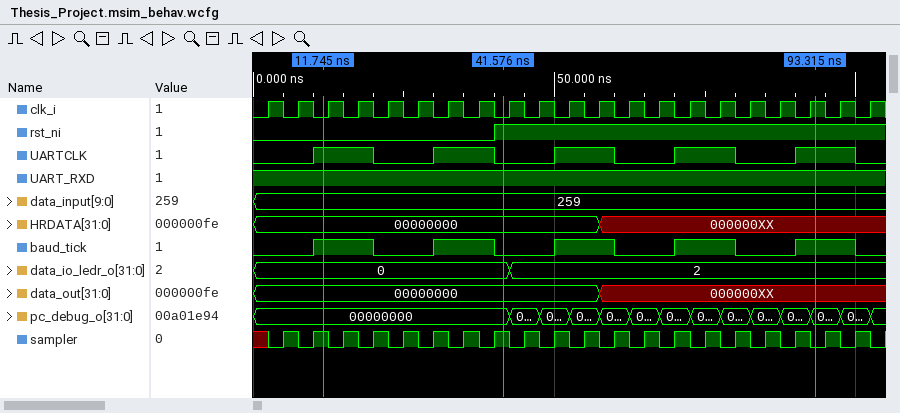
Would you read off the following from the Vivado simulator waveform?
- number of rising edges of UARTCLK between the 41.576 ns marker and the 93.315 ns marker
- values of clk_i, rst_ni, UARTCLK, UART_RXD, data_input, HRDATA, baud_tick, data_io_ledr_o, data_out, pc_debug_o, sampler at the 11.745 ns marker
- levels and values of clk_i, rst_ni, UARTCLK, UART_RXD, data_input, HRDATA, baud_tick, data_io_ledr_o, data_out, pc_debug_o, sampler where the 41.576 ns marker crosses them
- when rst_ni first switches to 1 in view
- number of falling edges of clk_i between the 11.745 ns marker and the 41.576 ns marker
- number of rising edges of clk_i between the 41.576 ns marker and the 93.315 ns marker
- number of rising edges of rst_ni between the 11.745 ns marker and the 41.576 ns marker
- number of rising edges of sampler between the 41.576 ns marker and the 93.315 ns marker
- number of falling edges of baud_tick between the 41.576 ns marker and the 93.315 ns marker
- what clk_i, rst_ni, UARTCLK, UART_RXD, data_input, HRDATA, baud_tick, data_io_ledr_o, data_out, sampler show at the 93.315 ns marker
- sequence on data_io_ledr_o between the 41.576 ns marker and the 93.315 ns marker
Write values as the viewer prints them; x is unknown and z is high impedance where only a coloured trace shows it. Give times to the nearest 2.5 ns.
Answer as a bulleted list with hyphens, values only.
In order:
- 3
- clk_i=0, rst_ni=0, UARTCLK=1, UART_RXD=1, data_input=259, HRDATA=00000000, baud_tick=1, data_io_ledr_o=0, data_out=00000000, pc_debug_o=00000000, sampler=1
- clk_i=0, rst_ni=1, UARTCLK=0, UART_RXD=1, data_input=259, HRDATA=00000000, baud_tick=0, data_io_ledr_o=0, data_out=00000000, pc_debug_o=00000000, sampler=1
- 40 ns
- 6
- 11
- 1
- 10
- 2
- clk_i=1, rst_ni=1, UARTCLK=1, UART_RXD=1, data_input=259, HRDATA=000000XX, baud_tick=1, data_io_ledr_o=2, data_out=000000XX, sampler=0
- 0, 2
